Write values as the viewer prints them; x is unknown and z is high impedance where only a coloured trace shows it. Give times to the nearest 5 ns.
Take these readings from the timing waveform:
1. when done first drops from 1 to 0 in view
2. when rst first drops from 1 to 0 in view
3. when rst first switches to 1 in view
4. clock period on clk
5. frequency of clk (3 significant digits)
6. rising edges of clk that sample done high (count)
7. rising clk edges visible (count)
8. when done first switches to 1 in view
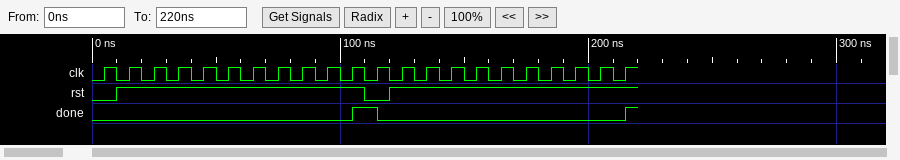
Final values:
115 ns
110 ns
10 ns
10 ns
100 MHz
1
22
105 ns
